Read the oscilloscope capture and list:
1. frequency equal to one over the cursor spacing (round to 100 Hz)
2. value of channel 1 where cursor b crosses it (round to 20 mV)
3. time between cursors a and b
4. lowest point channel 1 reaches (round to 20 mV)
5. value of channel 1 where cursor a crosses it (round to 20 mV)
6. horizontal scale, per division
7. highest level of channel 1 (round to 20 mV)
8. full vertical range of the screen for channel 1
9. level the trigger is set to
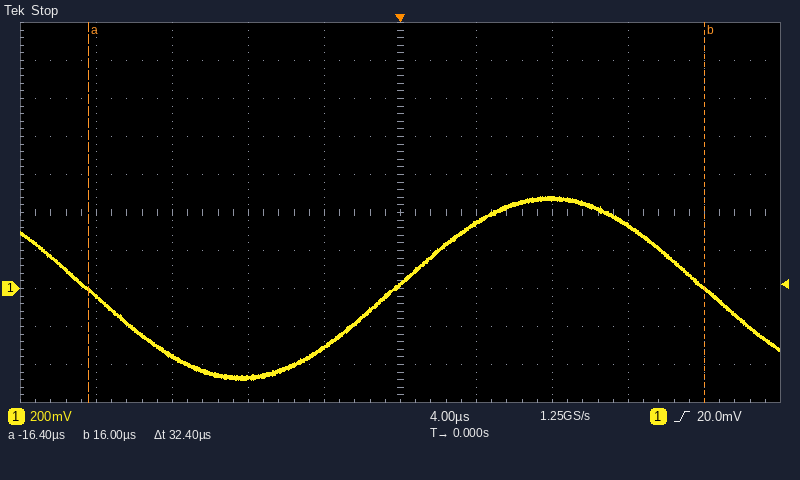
30.9 kHz
0 mV
32.4 µs
-480 mV
0 mV
4 µs
480 mV
2 V
20.0 mV
